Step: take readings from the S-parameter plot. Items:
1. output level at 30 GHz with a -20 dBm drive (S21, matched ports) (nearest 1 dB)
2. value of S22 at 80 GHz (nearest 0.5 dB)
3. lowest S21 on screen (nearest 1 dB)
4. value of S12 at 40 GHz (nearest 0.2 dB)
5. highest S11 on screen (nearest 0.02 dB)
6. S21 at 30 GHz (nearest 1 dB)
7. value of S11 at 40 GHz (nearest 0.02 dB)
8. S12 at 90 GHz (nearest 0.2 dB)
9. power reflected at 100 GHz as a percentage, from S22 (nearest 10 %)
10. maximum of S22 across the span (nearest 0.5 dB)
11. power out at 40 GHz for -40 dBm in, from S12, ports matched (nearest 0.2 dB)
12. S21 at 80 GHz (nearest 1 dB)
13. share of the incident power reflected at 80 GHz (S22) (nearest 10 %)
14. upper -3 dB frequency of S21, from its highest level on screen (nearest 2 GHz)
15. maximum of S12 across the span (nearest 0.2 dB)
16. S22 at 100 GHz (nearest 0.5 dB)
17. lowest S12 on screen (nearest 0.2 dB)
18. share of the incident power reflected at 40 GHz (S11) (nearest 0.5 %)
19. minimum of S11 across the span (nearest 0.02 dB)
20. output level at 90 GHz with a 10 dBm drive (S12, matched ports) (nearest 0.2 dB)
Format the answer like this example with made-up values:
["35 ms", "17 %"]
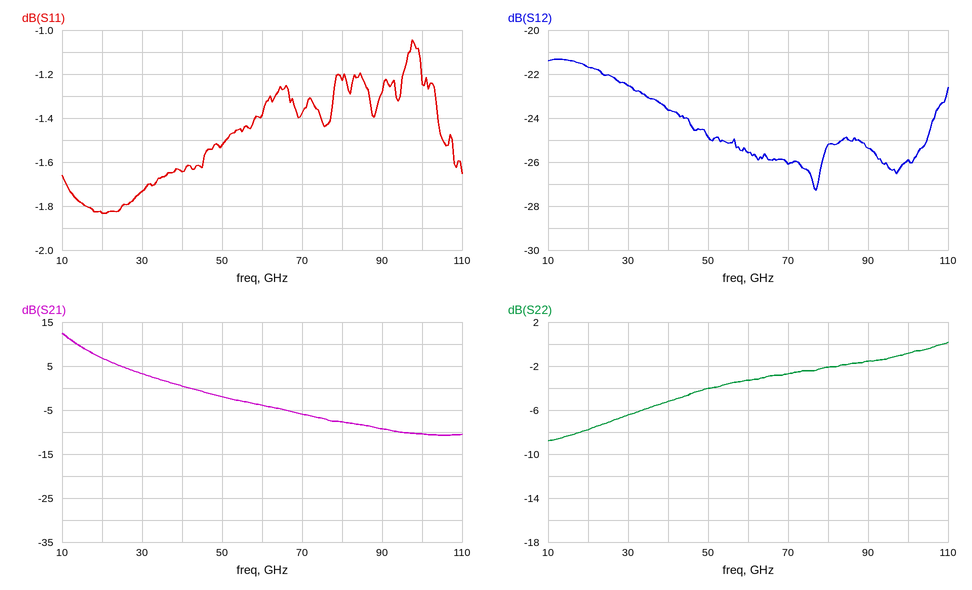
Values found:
["-17 dBm", "-2.0 dB", "-11 dB", "-23.6 dB", "-1.04 dB", "3 dB", "-1.64 dB", "-25.4 dB", "80 %", "0.0 dB", "-63.6 dBm", "-8 dB", "60 %", "14 GHz", "-21.4 dB", "-1.0 dB", "-27.2 dB", "68.5 %", "-1.84 dB", "-15.4 dBm"]
